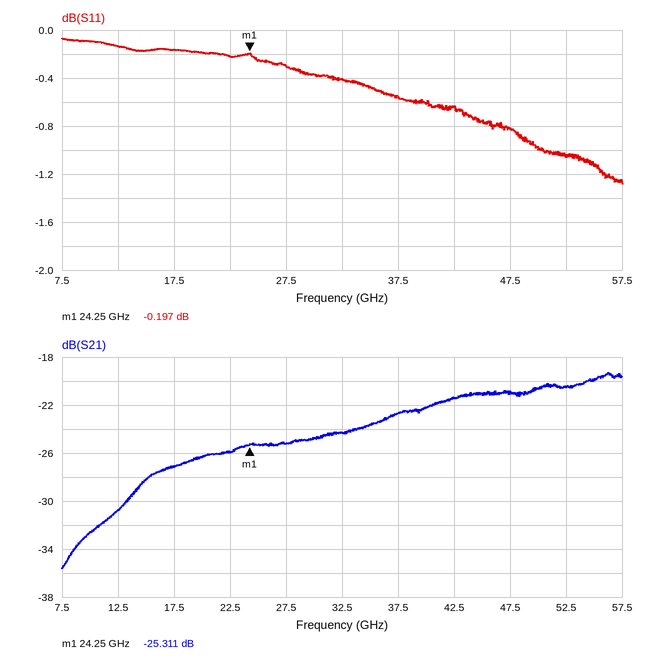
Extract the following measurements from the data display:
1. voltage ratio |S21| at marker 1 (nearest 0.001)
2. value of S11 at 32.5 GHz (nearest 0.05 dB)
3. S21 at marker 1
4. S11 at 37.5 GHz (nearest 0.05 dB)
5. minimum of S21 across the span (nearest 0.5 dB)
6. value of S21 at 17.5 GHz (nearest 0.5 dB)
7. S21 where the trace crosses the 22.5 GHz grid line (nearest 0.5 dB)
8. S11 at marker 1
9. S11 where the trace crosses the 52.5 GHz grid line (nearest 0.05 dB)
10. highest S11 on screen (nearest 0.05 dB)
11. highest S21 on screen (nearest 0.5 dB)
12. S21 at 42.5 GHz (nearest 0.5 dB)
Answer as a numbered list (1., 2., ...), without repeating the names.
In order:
1. 0.054
2. -0.40 dB
3. -25.311 dB
4. -0.55 dB
5. -35.5 dB
6. -27.0 dB
7. -26.0 dB
8. -0.197 dB
9. -1.05 dB
10. -0.05 dB
11. -19.5 dB
12. -21.5 dB
